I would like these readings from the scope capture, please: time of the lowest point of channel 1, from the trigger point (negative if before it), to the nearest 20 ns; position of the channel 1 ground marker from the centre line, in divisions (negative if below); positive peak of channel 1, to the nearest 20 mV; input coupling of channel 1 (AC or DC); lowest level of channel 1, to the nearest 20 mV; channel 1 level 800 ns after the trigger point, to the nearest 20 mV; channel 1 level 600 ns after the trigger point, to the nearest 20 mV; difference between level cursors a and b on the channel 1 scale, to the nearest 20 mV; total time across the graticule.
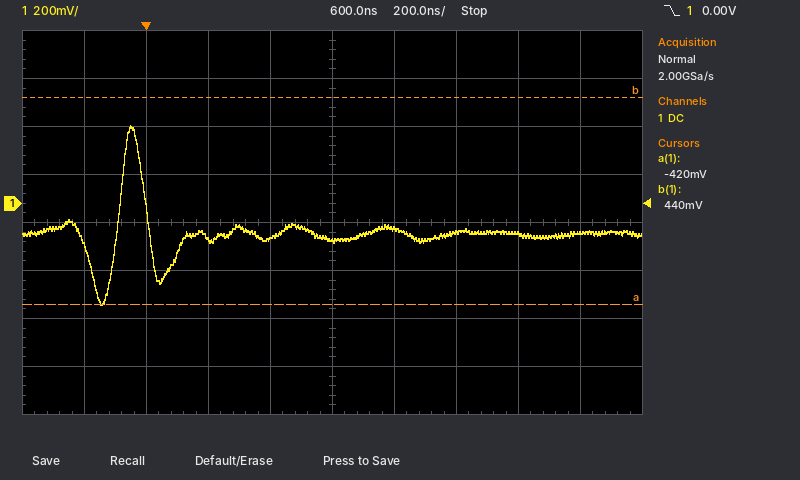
-140 ns
+0.4 div
320 mV
DC
-420 mV
-100 mV
-160 mV
860 mV
2 µs
